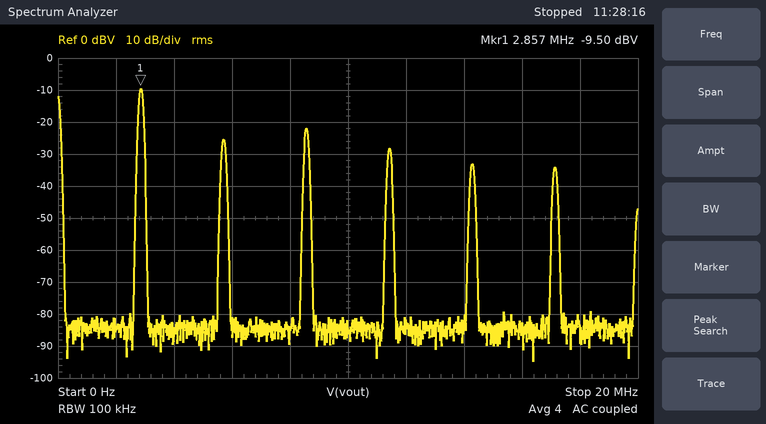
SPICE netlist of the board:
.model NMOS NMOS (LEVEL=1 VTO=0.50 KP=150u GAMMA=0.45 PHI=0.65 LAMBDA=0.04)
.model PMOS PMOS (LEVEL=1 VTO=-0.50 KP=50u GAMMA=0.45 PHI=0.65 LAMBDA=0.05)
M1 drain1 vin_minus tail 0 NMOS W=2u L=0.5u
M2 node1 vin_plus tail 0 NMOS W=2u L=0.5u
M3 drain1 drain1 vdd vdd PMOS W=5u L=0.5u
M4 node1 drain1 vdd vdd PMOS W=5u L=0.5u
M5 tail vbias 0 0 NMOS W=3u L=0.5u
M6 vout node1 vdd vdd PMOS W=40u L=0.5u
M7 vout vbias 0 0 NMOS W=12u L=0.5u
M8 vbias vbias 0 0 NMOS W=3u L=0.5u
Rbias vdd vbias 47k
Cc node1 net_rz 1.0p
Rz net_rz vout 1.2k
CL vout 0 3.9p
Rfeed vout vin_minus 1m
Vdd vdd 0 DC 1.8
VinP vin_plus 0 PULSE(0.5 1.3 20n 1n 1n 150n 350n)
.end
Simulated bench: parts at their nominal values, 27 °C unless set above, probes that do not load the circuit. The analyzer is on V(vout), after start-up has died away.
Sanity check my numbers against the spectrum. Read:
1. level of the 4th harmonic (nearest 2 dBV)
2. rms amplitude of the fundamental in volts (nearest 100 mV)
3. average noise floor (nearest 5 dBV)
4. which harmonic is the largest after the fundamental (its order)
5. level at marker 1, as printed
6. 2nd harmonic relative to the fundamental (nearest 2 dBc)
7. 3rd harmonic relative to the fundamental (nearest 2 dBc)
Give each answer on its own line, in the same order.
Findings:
-28 dBV
300 mV
-85 dBV
3
-9.50 dBV
-16 dBc
-12 dBc
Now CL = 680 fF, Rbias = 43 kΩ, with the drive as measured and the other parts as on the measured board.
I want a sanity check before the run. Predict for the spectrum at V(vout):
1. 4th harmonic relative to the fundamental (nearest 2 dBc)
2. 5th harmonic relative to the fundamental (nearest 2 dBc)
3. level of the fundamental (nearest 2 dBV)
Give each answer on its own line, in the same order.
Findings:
-18 dBc
-26 dBc
-10 dBV
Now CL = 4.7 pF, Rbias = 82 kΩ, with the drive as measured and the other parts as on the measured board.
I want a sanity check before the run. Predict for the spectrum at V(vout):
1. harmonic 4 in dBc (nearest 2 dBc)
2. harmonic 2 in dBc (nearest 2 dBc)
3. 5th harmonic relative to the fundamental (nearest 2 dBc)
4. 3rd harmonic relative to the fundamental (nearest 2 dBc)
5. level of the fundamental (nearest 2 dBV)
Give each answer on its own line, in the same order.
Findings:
-28 dBc
-22 dBc
-34 dBc
-18 dBc
-8 dBV
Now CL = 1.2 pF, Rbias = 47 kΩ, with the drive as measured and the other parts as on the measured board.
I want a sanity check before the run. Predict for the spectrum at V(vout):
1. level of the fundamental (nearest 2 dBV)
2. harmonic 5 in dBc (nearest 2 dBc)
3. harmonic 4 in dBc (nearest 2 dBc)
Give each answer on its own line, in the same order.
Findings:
-10 dBV
-26 dBc
-18 dBc
